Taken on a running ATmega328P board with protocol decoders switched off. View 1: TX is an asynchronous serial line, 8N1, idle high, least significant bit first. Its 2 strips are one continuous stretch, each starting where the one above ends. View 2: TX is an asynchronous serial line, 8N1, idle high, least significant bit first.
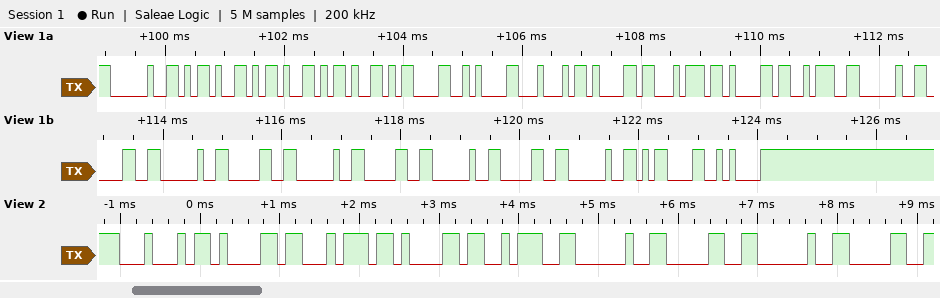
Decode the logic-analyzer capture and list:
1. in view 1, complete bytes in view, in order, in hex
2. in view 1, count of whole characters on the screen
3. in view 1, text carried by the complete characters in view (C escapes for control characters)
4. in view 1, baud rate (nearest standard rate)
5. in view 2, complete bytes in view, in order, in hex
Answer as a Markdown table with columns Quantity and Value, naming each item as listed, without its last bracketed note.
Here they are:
| Quantity | Value |
|---|---|
| in view 1, complete bytes in view, in order, in hex | 20 2D 2D 2D 0D 0A 44 61 74 61 3A 20 30 20 30 20 30 20 30 20 0D 0A |
| in view 1, count of whole characters on the screen | 22 |
| in view 1, text carried by the complete characters in view | " ---\r\nData: 0 0 0 0 \r\n" |
| in view 1, baud rate | 9600 baud |
| in view 2, complete bytes in view, in order, in hex | 44 61 74 61 3A 20 30 20 30 |
